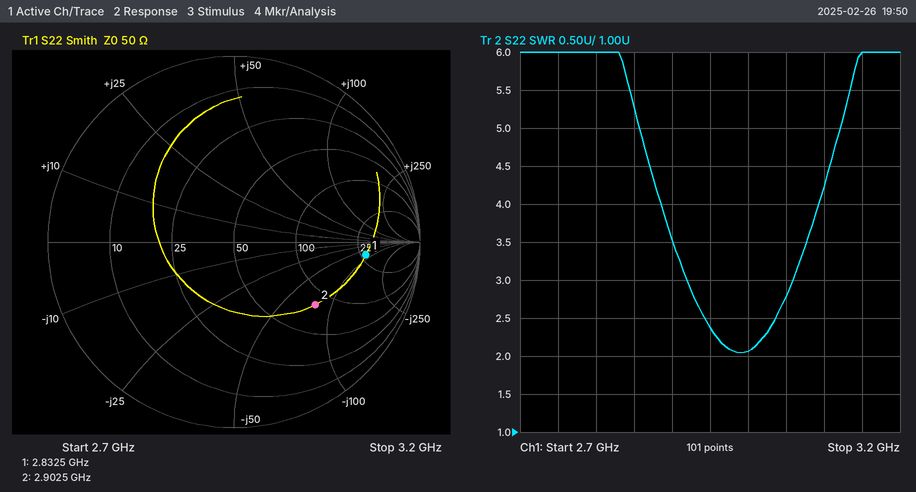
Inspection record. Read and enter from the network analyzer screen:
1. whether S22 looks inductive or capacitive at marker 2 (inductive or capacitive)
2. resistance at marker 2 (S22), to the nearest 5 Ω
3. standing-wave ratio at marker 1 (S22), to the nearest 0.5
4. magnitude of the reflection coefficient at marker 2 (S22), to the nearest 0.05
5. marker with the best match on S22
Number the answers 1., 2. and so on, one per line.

1. capacitive
2. 80 Ω
3. 6.0
4. 0.55
5. marker 2
